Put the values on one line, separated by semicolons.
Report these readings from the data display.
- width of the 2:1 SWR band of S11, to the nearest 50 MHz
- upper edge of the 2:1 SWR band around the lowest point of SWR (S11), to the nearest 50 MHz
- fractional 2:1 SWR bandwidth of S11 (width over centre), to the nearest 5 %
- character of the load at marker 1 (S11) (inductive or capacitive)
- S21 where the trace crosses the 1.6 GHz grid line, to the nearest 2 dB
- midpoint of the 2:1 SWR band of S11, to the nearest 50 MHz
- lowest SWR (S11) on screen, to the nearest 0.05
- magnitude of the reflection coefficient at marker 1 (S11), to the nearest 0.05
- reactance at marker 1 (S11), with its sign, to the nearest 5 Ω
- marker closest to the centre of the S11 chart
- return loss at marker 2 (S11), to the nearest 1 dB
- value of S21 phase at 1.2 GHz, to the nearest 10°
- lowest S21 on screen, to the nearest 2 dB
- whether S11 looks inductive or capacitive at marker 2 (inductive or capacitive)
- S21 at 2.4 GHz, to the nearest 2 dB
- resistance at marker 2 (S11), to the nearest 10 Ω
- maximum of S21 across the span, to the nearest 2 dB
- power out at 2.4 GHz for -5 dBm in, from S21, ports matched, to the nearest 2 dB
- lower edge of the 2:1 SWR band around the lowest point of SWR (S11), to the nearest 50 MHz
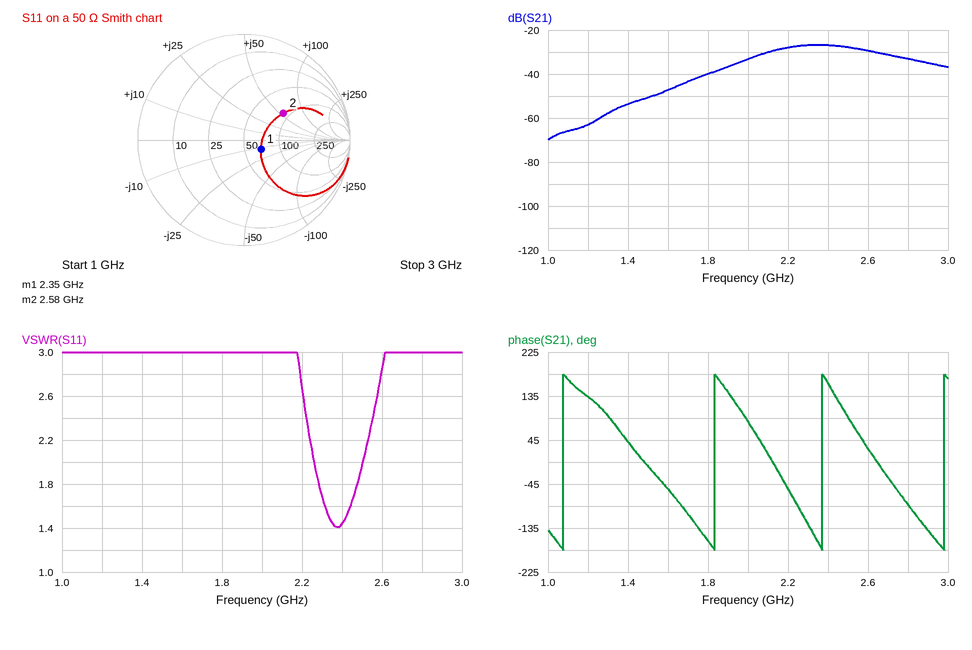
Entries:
250 MHz; 2.50 GHz; 10 %; capacitive; -48 dB; 2.40 GHz; 1.40; 0.20; -10 Ω; marker 1; 7 dB; 130°; -70 dB; inductive; -26 dB; 90 Ω; -26 dB; -32 dBm; 2.25 GHz
